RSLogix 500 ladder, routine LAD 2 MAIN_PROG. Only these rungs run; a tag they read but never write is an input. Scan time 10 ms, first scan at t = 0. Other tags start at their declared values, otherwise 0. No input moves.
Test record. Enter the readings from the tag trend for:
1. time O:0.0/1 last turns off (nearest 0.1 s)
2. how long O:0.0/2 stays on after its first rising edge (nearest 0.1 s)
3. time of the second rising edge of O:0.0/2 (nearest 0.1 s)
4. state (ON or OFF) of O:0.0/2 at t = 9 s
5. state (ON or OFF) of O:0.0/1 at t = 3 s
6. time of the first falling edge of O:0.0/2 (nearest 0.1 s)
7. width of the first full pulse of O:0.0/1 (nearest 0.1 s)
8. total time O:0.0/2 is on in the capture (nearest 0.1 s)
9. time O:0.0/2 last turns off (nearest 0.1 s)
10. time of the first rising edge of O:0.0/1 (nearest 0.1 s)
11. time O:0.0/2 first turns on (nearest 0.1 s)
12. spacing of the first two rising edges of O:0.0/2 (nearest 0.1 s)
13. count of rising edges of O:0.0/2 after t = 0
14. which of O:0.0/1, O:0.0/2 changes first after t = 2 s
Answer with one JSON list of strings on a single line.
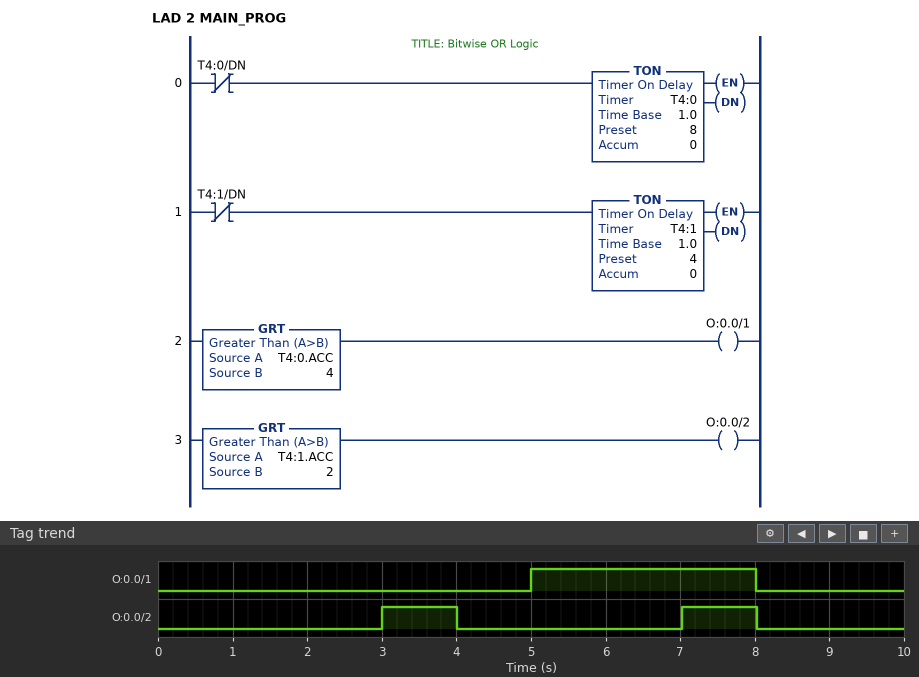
["8.0 s", "1.0 s", "7.0 s", "OFF", "OFF", "4.0 s", "3.0 s", "2.0 s", "8.0 s", "5.0 s", "3.0 s", "4.0 s", "2", "O:0.0/2"]
